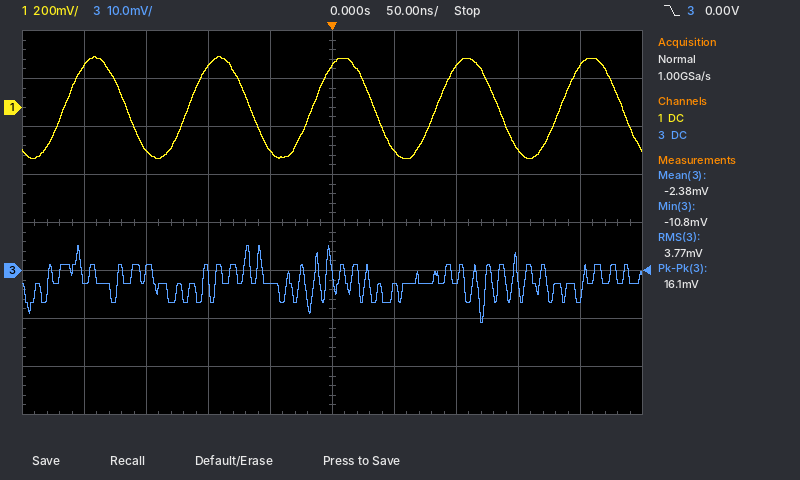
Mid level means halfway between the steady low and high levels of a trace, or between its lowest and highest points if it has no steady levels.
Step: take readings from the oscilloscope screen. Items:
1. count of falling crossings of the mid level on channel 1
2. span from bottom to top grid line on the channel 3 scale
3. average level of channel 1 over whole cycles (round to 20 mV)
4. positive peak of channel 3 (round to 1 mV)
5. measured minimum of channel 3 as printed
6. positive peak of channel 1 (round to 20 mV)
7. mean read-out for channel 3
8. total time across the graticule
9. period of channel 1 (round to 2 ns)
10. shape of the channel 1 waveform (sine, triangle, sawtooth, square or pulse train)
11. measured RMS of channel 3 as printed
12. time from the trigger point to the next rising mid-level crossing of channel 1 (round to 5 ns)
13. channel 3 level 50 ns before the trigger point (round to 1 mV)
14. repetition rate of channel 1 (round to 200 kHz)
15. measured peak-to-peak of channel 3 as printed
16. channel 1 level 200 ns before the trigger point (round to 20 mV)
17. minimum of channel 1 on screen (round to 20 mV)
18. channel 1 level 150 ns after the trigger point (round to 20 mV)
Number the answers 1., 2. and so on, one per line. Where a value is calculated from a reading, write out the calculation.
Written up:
1. 5
2. 80 mV
3. (220 mV + (-220 mV)) / 2 ≈ 0 mV
4. 5 mV
5. -10.8 mV
6. 220 mV
7. -2.38 mV
8. 500 ns
9. 100 ns
10. sine
11. 3.77 mV
12. 85 ns
13. -3 mV
14. 1 / 100 ns ≈ 10.0 MHz
15. 16.1 mV
16. 180 mV
17. -220 mV
18. -180 mV
